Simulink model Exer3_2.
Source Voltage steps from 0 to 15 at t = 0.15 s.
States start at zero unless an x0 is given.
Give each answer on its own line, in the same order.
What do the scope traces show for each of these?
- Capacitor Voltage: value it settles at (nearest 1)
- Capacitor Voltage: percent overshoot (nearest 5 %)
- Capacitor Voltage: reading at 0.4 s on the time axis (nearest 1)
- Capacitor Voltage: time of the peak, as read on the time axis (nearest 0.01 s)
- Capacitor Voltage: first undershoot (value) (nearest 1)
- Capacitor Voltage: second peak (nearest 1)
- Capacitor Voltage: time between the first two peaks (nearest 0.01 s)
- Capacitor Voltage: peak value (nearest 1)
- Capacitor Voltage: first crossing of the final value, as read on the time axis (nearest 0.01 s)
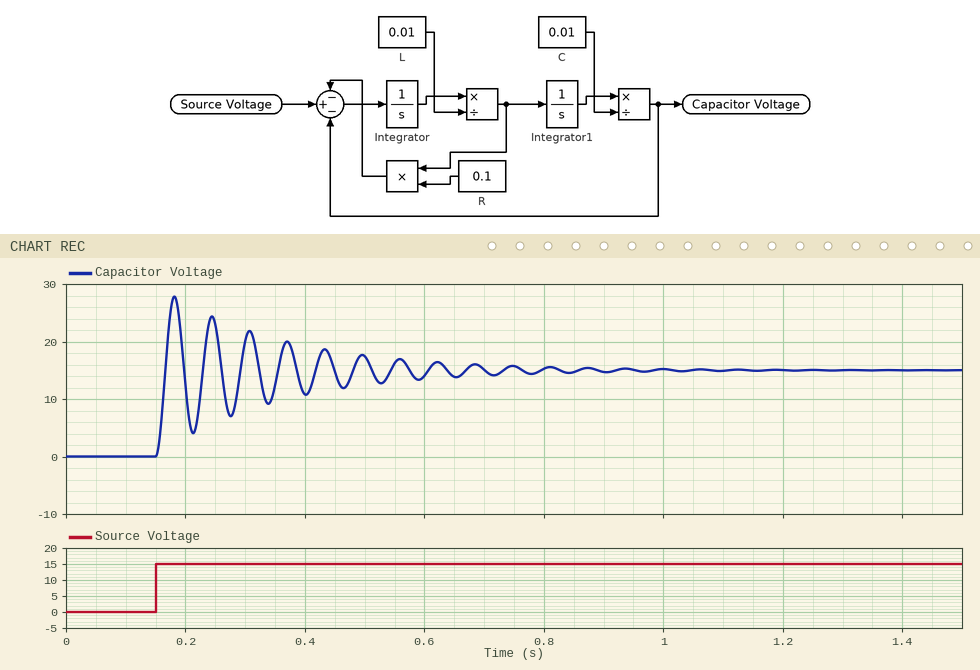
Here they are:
15
85 %
11
0.18 s
4
24
0.06 s
28
0.17 s
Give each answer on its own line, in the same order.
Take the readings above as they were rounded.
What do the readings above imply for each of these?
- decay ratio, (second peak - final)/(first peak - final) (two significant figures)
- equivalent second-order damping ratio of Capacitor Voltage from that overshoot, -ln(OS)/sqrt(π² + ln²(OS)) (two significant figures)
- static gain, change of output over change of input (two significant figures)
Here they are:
0.69
0.052
1.0
